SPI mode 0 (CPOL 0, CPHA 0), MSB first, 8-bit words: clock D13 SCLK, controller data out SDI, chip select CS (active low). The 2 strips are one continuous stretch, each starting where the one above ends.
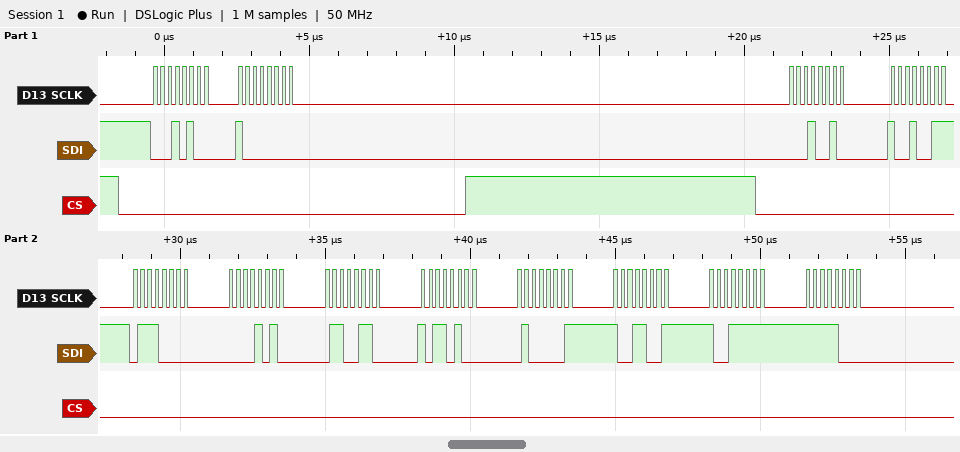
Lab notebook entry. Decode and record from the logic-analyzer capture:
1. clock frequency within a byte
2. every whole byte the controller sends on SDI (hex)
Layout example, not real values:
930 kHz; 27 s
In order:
4 MHz; 14 80 12 93 70 0A 66 B4 41 99 9F F8
